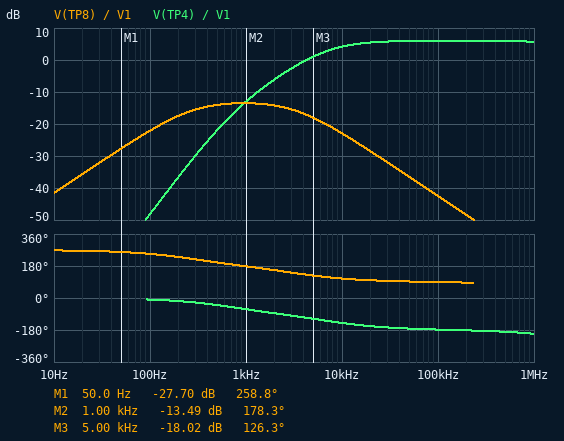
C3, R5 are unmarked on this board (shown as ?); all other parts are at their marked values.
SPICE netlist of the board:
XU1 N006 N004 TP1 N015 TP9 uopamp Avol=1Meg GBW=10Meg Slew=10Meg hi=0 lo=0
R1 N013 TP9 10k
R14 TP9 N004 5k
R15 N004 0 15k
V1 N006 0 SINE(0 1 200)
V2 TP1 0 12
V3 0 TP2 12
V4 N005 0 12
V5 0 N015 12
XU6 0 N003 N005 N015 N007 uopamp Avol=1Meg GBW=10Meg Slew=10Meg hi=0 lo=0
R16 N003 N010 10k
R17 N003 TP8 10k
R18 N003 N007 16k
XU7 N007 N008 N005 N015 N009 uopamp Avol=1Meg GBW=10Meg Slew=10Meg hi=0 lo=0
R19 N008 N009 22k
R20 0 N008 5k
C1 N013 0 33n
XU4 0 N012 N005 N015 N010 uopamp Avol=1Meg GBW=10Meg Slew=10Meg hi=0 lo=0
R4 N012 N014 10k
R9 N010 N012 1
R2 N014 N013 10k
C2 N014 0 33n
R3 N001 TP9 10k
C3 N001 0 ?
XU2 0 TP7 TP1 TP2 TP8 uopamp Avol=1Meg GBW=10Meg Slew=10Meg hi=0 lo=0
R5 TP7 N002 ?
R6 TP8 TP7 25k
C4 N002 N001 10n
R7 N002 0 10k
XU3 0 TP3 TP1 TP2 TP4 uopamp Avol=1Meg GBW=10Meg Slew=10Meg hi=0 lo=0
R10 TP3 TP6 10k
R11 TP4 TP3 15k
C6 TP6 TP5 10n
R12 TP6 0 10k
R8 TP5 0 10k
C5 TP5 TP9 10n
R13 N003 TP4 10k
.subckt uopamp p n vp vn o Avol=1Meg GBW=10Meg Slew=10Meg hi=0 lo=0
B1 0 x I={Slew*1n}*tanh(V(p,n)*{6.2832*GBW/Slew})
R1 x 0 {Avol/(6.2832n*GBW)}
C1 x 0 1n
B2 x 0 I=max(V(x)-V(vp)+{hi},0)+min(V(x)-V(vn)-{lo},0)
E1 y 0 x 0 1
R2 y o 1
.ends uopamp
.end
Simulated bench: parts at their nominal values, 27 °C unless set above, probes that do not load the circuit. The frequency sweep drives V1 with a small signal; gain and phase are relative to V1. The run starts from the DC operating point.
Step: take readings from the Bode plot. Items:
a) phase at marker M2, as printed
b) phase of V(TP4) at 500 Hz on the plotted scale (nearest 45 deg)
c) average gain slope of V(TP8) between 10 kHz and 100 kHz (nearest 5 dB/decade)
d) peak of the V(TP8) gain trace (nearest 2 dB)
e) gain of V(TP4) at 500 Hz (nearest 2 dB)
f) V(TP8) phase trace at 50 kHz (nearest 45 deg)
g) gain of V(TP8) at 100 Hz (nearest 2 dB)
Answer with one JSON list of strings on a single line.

["178.3 deg", "-45 deg", "-20 dB/decade", "-14 dB", "-22 dB", "90 deg", "-22 dB"]
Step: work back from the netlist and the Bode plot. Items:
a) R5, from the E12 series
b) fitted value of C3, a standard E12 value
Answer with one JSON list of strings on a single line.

["15 kΩ", "47 nF"]
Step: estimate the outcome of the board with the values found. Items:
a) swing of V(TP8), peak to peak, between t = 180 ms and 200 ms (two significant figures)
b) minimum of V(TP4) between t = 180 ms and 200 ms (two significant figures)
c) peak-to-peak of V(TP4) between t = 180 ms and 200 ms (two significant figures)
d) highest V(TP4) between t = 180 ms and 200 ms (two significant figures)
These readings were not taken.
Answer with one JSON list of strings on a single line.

["270 mV", "-15 mV", "30 mV", "15 mV"]
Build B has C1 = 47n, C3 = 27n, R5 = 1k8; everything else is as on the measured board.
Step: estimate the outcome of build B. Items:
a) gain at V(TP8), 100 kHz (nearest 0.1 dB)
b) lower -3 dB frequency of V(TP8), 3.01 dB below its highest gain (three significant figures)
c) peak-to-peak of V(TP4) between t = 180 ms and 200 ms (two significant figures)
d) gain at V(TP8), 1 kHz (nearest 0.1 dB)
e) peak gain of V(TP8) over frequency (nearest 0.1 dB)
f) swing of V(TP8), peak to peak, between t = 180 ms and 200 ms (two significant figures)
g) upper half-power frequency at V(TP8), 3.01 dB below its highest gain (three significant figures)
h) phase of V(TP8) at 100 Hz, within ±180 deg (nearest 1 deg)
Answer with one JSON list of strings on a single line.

["-19.3 dB", "403 Hz", "30 mV", "-3.2 dB", "-2.7 dB", "640 mV", "15.5 kHz", "-104 deg"]
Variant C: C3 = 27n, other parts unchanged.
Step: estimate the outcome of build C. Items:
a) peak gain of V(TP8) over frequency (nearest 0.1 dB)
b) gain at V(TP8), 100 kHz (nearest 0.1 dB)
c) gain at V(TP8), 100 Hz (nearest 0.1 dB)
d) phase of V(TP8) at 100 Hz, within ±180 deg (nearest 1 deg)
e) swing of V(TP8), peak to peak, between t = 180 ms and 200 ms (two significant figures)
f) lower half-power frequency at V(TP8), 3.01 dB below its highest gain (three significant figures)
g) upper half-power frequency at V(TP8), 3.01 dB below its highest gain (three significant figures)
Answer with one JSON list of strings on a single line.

["-10.2 dB", "-37.7 dB", "-21.8 dB", "-105 deg", "300 mV", "342 Hz", "4.57 kHz"]
